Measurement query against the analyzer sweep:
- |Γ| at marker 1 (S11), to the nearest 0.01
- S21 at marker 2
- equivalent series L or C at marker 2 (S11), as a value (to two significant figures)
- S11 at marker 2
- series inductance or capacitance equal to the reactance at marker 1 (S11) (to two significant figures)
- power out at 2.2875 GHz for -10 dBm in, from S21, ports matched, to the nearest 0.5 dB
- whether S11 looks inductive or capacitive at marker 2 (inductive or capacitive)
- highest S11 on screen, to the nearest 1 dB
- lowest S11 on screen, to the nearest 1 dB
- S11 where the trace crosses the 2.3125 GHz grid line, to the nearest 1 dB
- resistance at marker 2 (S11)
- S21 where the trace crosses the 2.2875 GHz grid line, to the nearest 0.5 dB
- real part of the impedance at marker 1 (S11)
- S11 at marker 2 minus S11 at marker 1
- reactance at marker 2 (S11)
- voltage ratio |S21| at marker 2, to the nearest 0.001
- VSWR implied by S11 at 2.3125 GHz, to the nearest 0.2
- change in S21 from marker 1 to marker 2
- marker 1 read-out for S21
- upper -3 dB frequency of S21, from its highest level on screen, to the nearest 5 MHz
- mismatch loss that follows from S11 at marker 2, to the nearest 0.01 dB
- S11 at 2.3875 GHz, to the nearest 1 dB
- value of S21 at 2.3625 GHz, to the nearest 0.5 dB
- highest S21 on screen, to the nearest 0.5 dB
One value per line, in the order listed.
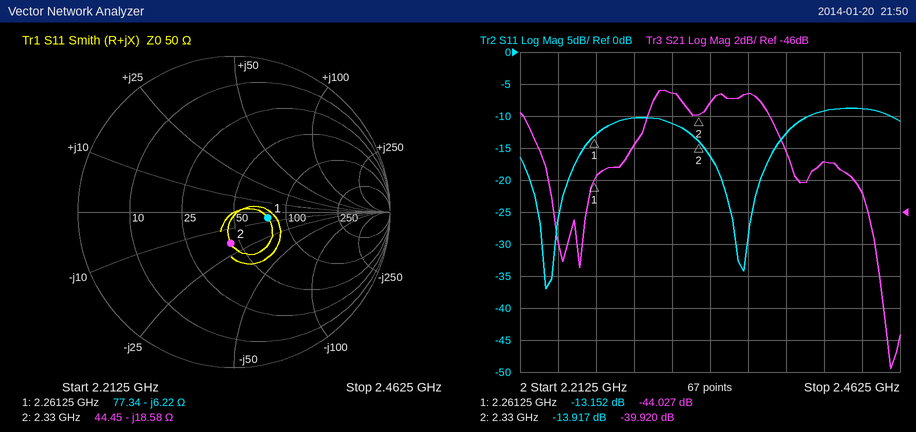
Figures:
0.22
-39.920 dB
3.7 pF
-13.917 dB
11 pF
-52.0 dBm
capacitive
-9 dB
-37 dB
-11 dB
44.45 Ω
-42.0 dB
77.34 Ω
-0.765 dB
-18.58 Ω
0.010
1.8
4.107 dB
-44.027 dB
2.385 GHz
0.18 dB
-13 dB
-38.5 dB
-38.5 dB
